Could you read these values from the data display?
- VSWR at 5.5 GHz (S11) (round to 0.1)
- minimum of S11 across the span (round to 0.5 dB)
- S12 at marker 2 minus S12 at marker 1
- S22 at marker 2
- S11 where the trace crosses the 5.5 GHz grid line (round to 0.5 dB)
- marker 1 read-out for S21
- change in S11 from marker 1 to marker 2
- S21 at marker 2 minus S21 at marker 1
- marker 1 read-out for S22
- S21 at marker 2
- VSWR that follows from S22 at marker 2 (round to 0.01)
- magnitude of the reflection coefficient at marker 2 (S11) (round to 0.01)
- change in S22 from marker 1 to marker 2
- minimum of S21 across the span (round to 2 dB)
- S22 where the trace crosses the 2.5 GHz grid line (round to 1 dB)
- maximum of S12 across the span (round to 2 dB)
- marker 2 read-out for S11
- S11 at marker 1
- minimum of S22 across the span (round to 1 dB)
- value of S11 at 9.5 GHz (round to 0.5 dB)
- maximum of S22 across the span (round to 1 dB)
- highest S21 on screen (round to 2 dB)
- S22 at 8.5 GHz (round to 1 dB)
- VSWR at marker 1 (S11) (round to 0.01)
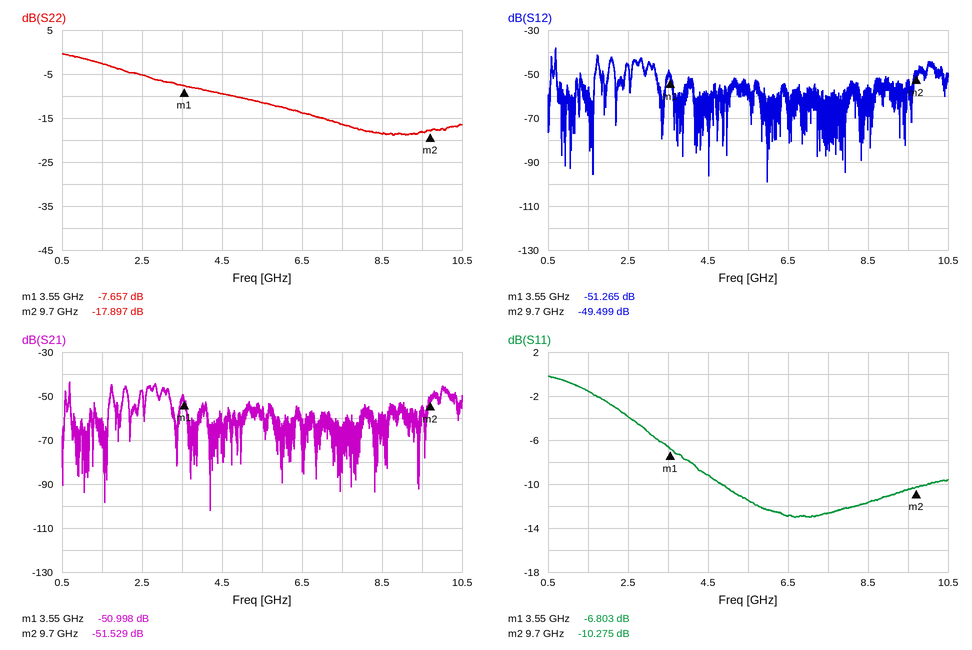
1.7
-13.0 dB
1.766 dB
-17.897 dB
-11.5 dB
-50.998 dB
-3.472 dB
-0.531 dB
-7.657 dB
-51.529 dB
1.29
0.31
-10.240 dB
-102 dB
-5 dB
-38 dB
-10.275 dB
-6.803 dB
-19 dB
-10.5 dB
0 dB
-44 dB
-19 dB
2.68
